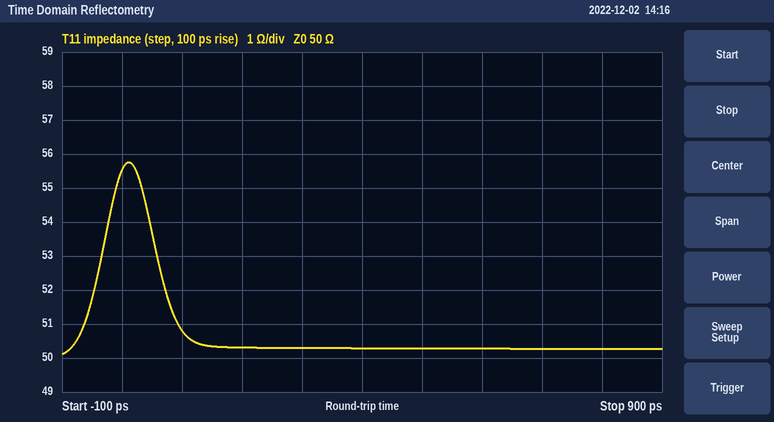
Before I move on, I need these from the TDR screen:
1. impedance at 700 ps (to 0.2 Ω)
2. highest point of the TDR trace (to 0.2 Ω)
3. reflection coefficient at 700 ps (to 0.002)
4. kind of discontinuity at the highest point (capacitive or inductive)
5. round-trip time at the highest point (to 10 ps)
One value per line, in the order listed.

50.2 Ω
55.8 Ω
+0.002
inductive
10 ps
